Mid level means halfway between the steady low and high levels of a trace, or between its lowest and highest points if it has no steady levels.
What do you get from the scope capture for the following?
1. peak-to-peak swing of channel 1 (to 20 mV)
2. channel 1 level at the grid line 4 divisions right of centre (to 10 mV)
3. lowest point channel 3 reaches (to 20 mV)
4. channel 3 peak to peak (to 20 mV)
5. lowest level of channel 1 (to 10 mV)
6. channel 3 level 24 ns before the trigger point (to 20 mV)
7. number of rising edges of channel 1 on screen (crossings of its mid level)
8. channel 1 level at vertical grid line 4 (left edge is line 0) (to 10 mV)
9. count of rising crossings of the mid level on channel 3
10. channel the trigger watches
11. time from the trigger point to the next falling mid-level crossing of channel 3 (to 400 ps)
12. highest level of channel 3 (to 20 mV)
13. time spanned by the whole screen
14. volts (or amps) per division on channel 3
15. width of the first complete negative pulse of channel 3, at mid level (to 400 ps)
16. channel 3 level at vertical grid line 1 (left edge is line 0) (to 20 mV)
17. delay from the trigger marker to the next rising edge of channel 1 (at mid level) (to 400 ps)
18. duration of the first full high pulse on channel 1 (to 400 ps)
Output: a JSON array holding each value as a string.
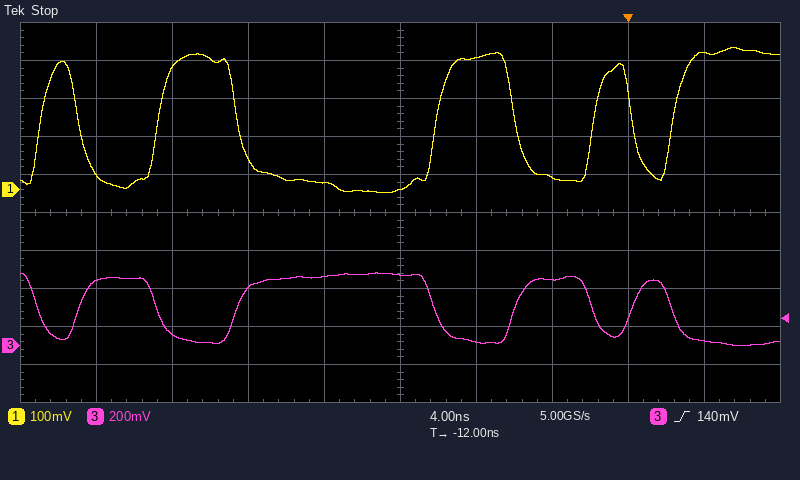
["380 mV", "360 mV", "0 mV", "380 mV", "-10 mV", "60 mV", "5", "20 mV", "4", "channel 3", "2.4 ns", "380 mV", "40 ns", "200 mV", "2.0 ns", "340 mV", "2.4 ns", "2.0 ns"]
